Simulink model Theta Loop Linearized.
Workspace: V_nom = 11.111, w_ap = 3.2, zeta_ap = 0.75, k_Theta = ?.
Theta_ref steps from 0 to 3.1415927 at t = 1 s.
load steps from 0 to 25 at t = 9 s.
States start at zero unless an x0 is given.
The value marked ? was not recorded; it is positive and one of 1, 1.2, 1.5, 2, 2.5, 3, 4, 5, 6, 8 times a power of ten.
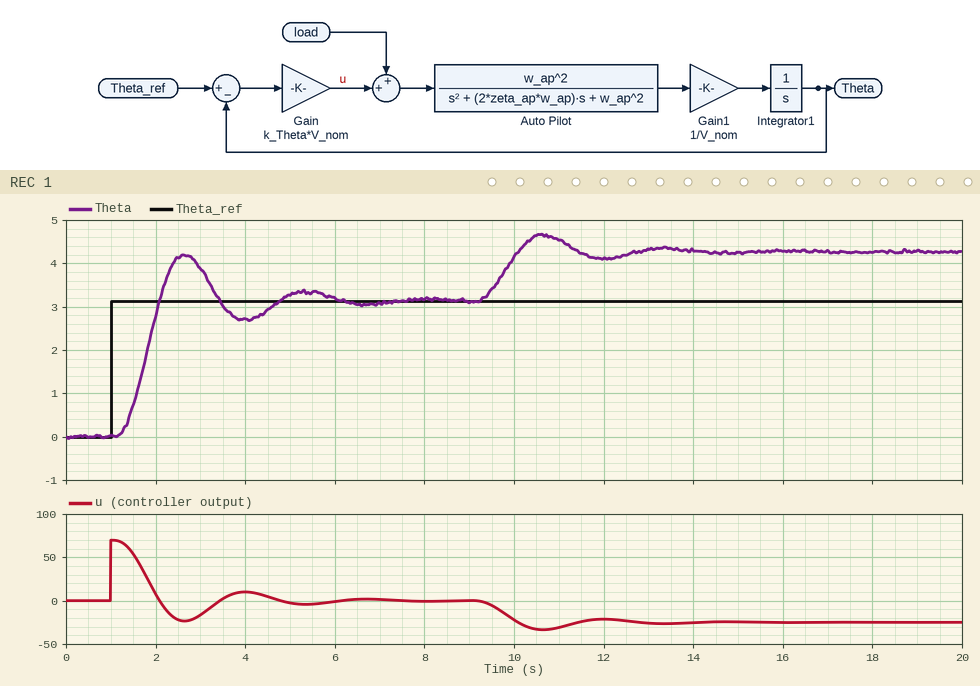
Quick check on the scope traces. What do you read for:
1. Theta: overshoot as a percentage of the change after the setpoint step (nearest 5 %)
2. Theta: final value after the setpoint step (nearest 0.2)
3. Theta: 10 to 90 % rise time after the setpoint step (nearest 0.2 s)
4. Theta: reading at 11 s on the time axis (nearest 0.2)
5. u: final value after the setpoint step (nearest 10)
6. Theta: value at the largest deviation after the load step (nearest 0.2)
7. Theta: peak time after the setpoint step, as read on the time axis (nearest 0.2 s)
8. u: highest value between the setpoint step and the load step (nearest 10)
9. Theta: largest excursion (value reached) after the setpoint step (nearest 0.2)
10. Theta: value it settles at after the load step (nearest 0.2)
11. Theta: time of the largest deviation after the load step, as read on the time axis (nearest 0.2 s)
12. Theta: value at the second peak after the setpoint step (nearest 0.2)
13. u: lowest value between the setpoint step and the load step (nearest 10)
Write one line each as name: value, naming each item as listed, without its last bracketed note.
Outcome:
Theta: overshoot as a percentage of the change after the setpoint step: 35 %
Theta: final value after the setpoint step: 3.2
Theta: 10 to 90 % rise time after the setpoint step: 0.6 s
Theta: reading at 11 s on the time axis: 4.6
u: final value after the setpoint step: 0
Theta: value at the largest deviation after the load step: 4.6
Theta: peak time after the setpoint step, as read on the time axis: 2.6 s
u: highest value between the setpoint step and the load step: 70
Theta: largest excursion (value reached) after the setpoint step: 4.2
Theta: value it settles at after the load step: 4.2
Theta: time of the largest deviation after the load step, as read on the time axis: 10.6 s
Theta: value at the second peak after the setpoint step: 3.4
u: lowest value between the setpoint step and the load step: -20
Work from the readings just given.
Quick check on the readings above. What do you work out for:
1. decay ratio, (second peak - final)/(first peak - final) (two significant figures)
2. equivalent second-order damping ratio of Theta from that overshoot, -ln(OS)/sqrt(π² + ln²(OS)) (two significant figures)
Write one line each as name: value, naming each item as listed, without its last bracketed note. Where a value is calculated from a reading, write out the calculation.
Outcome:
decay ratio, (second peak - final)/(first peak - final): (3.4 - 3.2) / (4.2 - 3.2) = 0.20
equivalent second-order damping ratio of Theta from that overshoot, -ln(OS)/sqrt(π² + ln²(OS)): ln(0.35) = -1.050; 1.050 / sqrt(9.870 + 1.102) = 0.32
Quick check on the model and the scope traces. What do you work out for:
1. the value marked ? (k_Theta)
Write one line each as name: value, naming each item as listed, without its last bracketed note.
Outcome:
the value marked ?: 2
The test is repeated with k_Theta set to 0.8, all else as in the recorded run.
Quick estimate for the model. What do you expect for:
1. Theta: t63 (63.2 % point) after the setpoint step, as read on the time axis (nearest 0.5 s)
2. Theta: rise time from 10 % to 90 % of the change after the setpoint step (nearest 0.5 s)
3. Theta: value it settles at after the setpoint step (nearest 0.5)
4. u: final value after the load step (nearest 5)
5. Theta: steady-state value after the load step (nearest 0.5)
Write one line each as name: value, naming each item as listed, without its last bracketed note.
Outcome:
Theta: t63 (63.2 % point) after the setpoint step, as read on the time axis: 2.5 s
Theta: rise time from 10 % to 90 % of the change after the setpoint step: 1.5 s
Theta: value it settles at after the setpoint step: 3.0
u: final value after the load step: -25
Theta: steady-state value after the load step: 6.0
